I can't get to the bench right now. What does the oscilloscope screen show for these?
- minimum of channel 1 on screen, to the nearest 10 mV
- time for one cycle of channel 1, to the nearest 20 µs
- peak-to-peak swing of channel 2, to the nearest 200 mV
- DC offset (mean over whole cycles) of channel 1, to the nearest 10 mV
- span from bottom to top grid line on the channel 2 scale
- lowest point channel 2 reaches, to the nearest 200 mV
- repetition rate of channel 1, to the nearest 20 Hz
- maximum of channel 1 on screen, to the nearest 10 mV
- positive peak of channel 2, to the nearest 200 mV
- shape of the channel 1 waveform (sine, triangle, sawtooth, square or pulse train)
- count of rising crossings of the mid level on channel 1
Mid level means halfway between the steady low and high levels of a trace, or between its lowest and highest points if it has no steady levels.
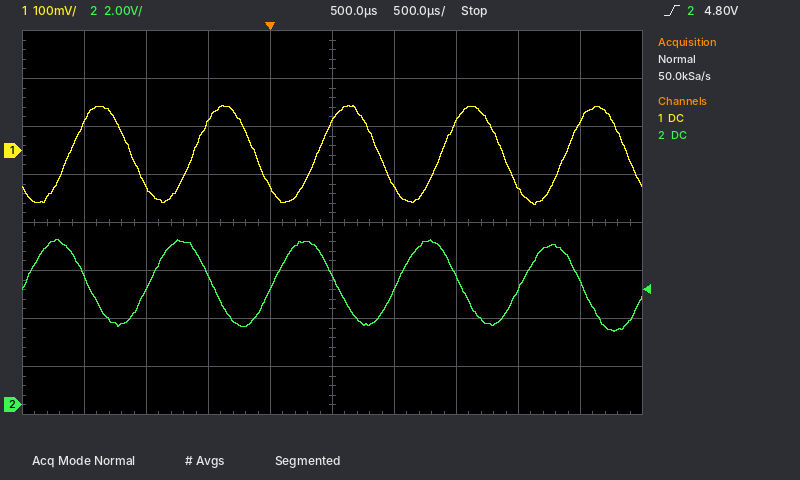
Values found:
-110 mV
1.00 ms
3.8 V
-10 mV
16 V
3.0 V
1.00 kHz
90 mV
6.8 V
sine
5
